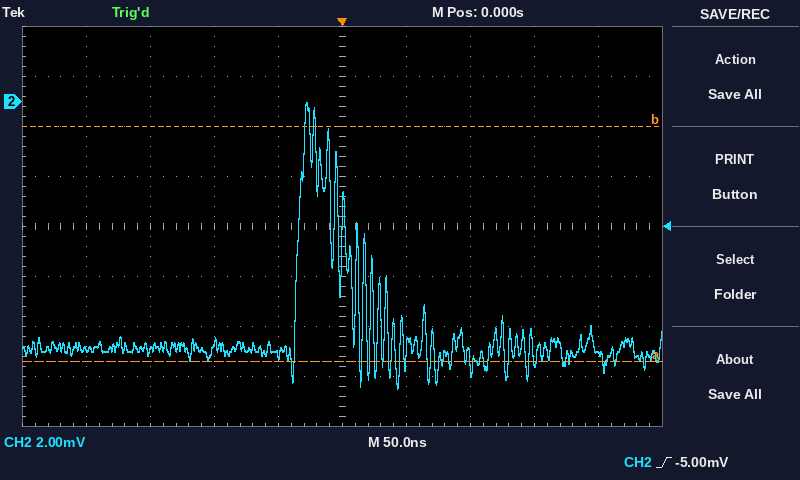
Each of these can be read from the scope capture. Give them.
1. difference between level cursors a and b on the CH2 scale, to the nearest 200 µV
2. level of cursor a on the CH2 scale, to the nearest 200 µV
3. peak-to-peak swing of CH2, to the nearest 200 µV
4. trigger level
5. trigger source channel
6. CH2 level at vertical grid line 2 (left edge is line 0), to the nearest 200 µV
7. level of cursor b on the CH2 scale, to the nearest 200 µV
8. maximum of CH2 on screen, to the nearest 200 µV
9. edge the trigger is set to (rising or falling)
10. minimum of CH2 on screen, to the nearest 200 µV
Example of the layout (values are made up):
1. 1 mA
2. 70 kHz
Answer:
1. 9.4 mV
2. -10.4 mV
3. 11.4 mV
4. -5.00 mV
5. CH2
6. -10.0 mV
7. -1.0 mV
8. 0.0 mV
9. rising
10. -11.4 mV
